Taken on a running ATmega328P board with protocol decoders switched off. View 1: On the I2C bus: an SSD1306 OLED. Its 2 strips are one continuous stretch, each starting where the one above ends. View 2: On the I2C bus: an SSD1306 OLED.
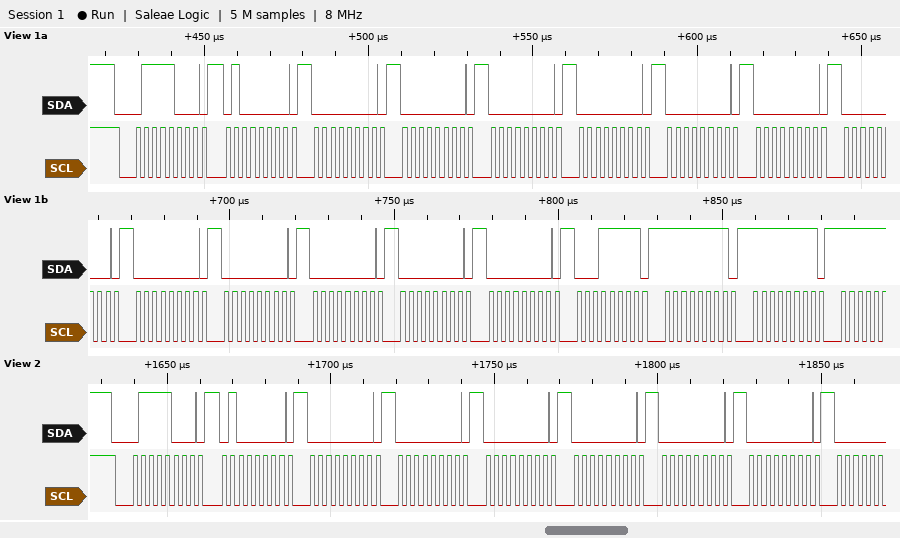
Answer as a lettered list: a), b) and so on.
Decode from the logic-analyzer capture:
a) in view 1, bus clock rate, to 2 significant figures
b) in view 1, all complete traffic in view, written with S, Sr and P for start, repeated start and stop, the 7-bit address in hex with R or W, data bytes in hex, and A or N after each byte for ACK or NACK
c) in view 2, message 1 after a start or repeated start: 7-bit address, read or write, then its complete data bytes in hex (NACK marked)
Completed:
a) 400 kHz
b) S 3CW A 40 A 00 A 00 A 00 A 00 A 00 A 00 A 00 A 00 A 00 A 00 A 00 A 00 A 1F A FF A FF A
c) 0x3C write: 40 00 00 00 00 00 00
